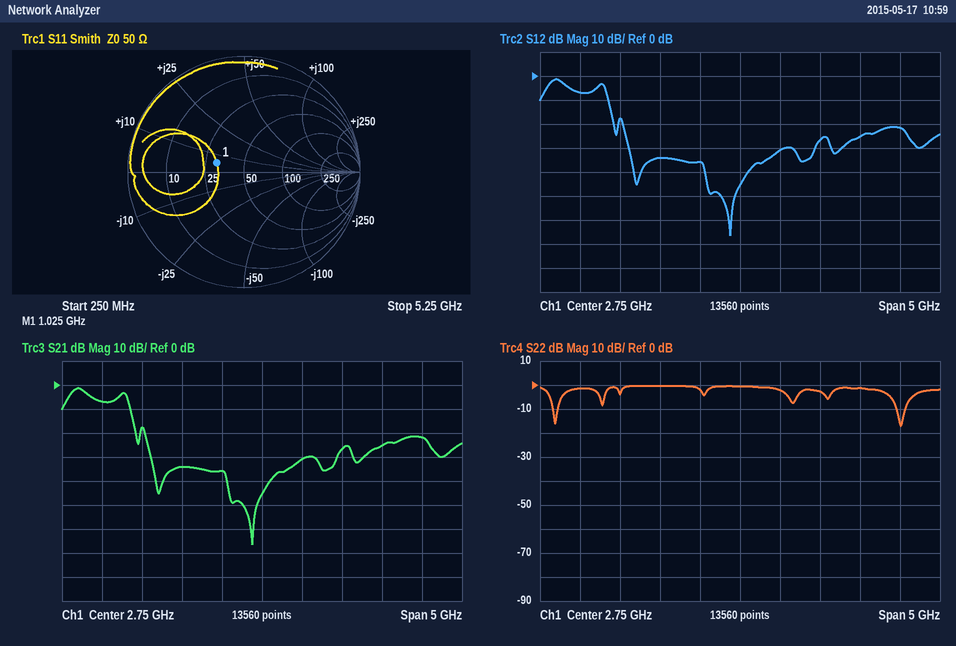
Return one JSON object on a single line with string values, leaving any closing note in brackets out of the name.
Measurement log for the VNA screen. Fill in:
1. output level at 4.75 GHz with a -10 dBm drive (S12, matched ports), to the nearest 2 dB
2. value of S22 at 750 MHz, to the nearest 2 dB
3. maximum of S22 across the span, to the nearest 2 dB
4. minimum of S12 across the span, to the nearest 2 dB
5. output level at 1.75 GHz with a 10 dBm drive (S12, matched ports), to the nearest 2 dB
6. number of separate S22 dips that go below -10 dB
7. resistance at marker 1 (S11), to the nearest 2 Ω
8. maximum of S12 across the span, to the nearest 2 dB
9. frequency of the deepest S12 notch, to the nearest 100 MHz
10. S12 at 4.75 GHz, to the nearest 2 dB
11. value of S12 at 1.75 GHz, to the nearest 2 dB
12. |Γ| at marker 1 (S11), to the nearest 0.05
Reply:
{"output level at 4.75 GHz with a -10 dBm drive (S12, matched ports), to the nearest 2 dB": "-32 dBm", "value of S22 at 750 MHz, to the nearest 2 dB": "-2 dB", "maximum of S22 across the span, to the nearest 2 dB": "0 dB", "minimum of S12 across the span, to the nearest 2 dB": "-66 dB", "output level at 1.75 GHz with a 10 dBm drive (S12, matched ports), to the nearest 2 dB": "-24 dBm", "number of separate S22 dips that go below -10 dB": "2", "resistance at marker 1 (S11), to the nearest 2 Ω": "30 Ω", "maximum of S12 across the span, to the nearest 2 dB": "-2 dB", "frequency of the deepest S12 notch, to the nearest 100 MHz": "2.6 GHz", "S12 at 4.75 GHz, to the nearest 2 dB": "-22 dB", "value of S12 at 1.75 GHz, to the nearest 2 dB": "-34 dB", "|Γ| at marker 1 (S11), to the nearest 0.05": "0.25"}
